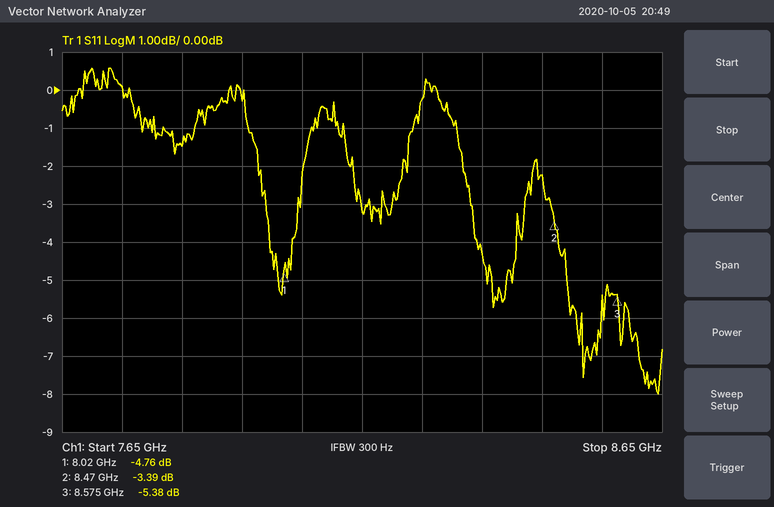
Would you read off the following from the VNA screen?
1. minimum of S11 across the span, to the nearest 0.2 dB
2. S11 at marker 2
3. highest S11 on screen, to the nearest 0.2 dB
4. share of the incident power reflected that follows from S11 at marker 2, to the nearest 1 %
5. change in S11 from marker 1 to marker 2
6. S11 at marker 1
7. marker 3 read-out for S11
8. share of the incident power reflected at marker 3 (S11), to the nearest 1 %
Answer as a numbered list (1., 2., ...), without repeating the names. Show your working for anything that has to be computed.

1. -8.0 dB
2. -3.39 dB
3. 0.6 dB
4. 10^(-3.39/10) ≈ 46 %
5. -3.39 − (-4.76) = 1.37 dB
6. -4.76 dB
7. -5.38 dB
8. 10^(-5.38/10) ≈ 29 %
